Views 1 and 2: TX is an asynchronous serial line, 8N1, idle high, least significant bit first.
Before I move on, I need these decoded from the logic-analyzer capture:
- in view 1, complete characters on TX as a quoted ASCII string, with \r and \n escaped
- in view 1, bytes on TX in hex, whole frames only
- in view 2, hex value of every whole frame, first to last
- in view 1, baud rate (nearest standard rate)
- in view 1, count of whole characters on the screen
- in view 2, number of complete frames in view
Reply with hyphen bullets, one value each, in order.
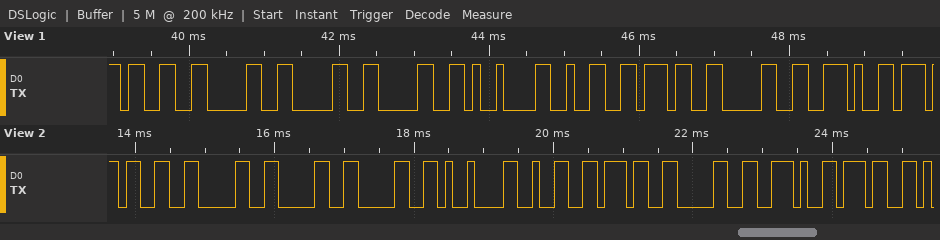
- "3000\t270."
- 33 30 30 30 09 32 37 30 2E
- 33 30 30 30 09 32 37 30 2E 37
- 9600 baud
- 9
- 10
